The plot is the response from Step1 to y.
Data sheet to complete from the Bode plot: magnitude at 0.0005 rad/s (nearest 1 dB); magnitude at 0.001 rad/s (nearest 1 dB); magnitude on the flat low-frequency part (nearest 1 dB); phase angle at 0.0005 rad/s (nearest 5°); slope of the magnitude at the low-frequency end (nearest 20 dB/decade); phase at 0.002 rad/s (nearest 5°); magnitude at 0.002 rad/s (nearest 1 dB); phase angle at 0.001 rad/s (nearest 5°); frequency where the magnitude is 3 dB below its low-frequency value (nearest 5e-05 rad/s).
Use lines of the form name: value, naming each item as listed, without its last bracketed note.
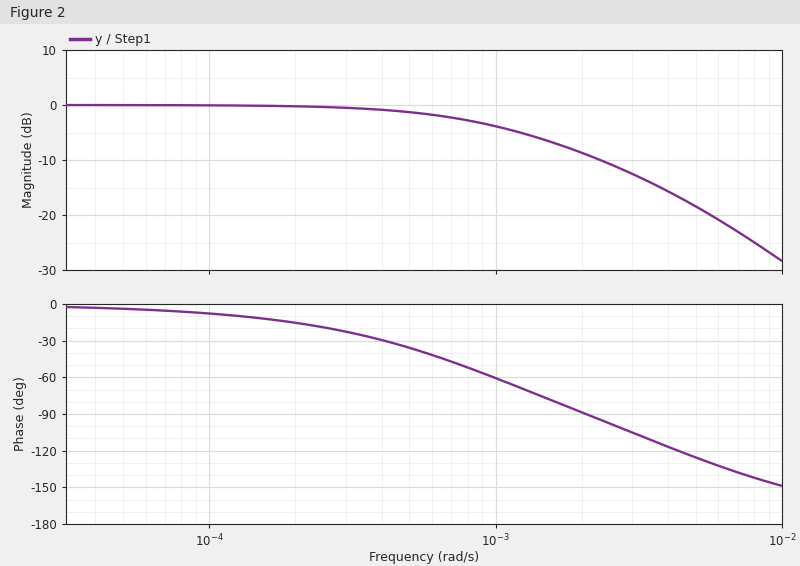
magnitude at 0.0005 rad/s: -1 dB
magnitude at 0.001 rad/s: -4 dB
magnitude on the flat low-frequency part: 0 dB
phase angle at 0.0005 rad/s: -35°
slope of the magnitude at the low-frequency end: 0 dB/decade
phase at 0.002 rad/s: -90°
magnitude at 0.002 rad/s: -9 dB
phase angle at 0.001 rad/s: -60°
frequency where the magnitude is 3 dB below its low-frequency value: 0.00085 rad/s
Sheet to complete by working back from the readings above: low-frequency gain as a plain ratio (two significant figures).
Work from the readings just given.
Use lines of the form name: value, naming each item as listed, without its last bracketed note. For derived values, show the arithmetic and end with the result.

low-frequency gain as a plain ratio: 10^(0 / 20) = 1.0
